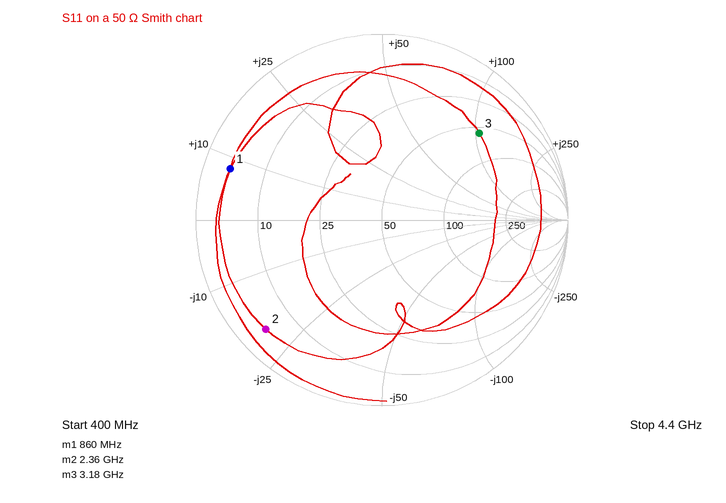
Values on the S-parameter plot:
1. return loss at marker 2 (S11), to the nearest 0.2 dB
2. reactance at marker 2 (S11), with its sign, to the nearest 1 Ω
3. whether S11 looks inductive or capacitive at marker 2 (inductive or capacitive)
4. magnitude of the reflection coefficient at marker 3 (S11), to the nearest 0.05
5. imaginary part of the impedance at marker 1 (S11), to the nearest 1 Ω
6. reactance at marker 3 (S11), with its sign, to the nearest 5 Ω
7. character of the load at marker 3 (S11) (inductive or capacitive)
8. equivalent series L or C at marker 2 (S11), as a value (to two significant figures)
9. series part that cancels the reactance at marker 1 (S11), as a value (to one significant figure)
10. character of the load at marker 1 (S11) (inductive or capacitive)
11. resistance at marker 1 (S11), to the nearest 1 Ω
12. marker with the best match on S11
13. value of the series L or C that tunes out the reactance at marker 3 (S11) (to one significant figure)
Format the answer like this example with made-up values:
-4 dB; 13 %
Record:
1.4 dB; -20 Ω; capacitive; 0.70; +8 Ω; +105 Ω; inductive; 3.4 pF; 20 pF; inductive; 4 Ω; marker 3; 500 fF
